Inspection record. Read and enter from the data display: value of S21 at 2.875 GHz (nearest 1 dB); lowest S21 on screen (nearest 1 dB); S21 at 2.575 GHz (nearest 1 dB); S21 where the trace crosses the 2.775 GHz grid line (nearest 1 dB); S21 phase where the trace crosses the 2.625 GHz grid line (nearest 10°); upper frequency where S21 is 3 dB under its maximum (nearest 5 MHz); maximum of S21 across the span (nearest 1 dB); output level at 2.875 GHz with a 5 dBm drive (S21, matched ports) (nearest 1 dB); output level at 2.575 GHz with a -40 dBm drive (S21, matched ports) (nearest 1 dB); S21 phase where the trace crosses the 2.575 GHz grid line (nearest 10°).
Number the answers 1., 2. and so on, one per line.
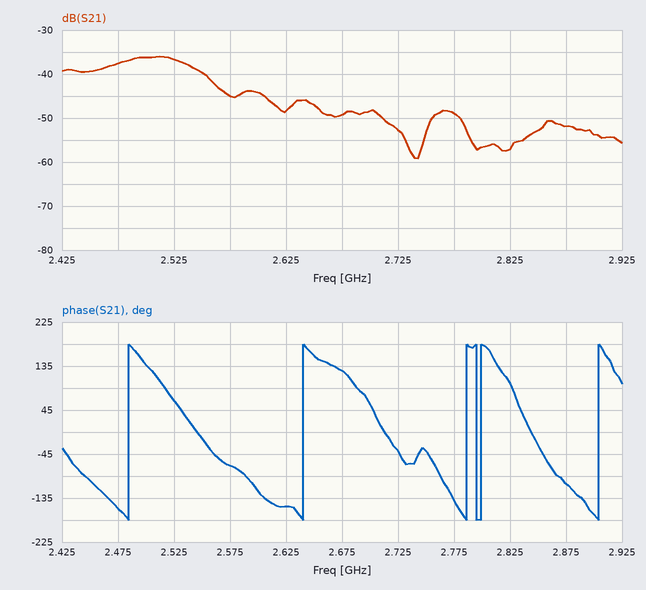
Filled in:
1. -52 dB
2. -59 dB
3. -45 dB
4. -49 dB
5. -150°
6. 2.545 GHz
7. -36 dB
8. -47 dBm
9. -85 dBm
10. -70°
